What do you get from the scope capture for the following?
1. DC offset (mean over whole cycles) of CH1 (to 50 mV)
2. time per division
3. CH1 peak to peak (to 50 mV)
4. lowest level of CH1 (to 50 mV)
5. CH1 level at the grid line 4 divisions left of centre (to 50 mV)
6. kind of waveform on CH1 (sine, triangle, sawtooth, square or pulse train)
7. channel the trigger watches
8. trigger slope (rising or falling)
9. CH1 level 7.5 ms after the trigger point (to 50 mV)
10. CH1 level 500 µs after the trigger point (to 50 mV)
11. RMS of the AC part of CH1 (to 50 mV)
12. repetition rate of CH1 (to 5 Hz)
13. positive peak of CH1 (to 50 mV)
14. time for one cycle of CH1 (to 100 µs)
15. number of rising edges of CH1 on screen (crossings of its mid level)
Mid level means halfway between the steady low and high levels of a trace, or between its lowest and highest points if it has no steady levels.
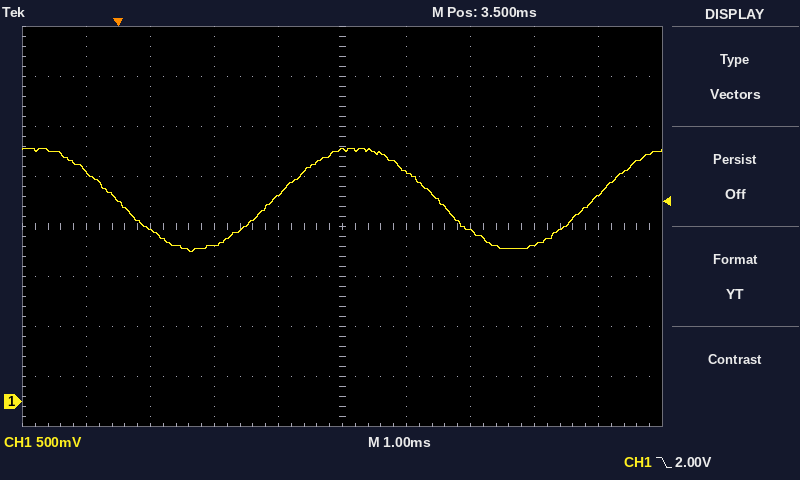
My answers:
2.05 V
1 ms
1.05 V
1.50 V
2.30 V
sine
CH1
falling
2.05 V
1.70 V
350 mV
200 Hz
2.55 V
5.0 ms
2
